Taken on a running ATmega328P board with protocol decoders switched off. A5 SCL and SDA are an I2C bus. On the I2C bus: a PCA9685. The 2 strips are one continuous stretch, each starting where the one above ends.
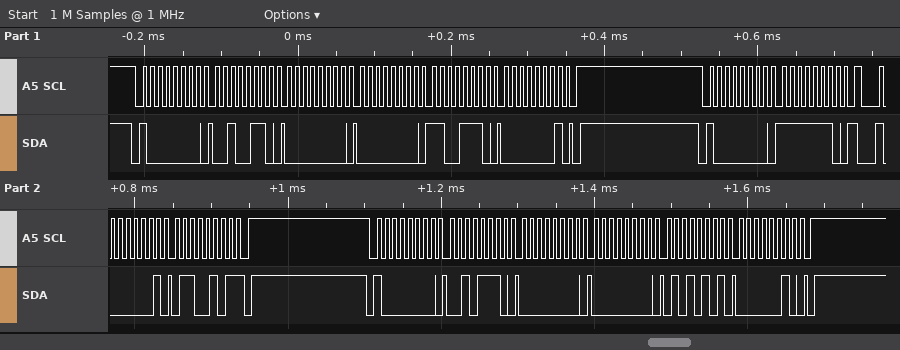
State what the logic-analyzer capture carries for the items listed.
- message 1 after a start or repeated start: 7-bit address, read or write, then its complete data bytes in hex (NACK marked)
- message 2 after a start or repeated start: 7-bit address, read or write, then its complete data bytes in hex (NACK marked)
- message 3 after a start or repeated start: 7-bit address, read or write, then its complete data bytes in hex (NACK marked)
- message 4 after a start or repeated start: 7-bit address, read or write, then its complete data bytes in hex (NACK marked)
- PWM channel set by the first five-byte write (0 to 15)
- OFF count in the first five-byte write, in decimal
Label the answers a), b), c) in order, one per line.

a) 0x40 write: 26 00 00 CE 01
b) 0x40 write: FE
c) 0x40 read: 65 NACK
d) 0x40 write: 2E 00 00 55 02
e) 8
f) 462
